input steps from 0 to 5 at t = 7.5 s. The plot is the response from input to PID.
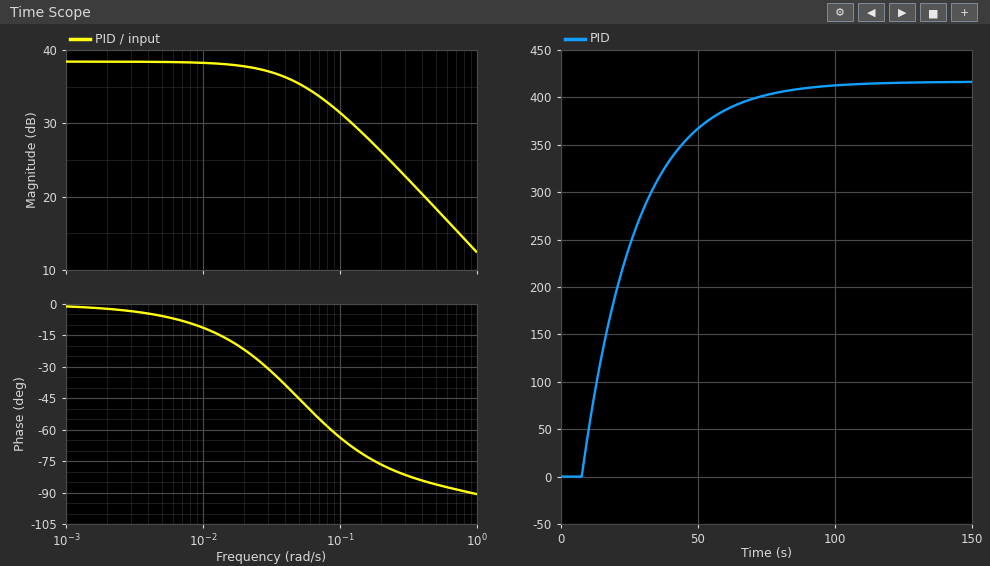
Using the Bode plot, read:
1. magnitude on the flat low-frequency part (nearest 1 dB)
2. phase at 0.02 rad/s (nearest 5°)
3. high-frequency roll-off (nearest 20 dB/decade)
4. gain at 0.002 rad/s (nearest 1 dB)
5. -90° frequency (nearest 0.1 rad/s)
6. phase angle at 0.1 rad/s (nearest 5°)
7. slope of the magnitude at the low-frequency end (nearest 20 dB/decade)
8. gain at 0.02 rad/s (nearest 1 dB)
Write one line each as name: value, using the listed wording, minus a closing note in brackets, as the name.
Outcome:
magnitude on the flat low-frequency part: 38 dB
phase at 0.02 rad/s: -20°
high-frequency roll-off: -20 dB/decade
gain at 0.002 rad/s: 38 dB
-90° frequency: 0.9 rad/s
phase angle at 0.1 rad/s: -65°
slope of the magnitude at the low-frequency end: 0 dB/decade
gain at 0.02 rad/s: 38 dB
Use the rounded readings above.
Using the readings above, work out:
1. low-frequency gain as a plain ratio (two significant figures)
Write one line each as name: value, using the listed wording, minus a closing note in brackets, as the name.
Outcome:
low-frequency gain as a plain ratio: 79
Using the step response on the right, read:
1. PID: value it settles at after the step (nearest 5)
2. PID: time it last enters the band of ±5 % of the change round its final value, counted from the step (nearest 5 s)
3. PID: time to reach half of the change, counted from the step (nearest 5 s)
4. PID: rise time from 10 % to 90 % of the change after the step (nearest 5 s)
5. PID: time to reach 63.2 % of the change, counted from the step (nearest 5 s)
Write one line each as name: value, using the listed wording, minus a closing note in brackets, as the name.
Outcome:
PID: value it settles at after the step: 415
PID: time it last enters the band of ±5 % of the change round its final value, counted from the step: 60 s
PID: time to reach half of the change, counted from the step: 15 s
PID: rise time from 10 % to 90 % of the change after the step: 45 s
PID: time to reach 63.2 % of the change, counted from the step: 20 s
